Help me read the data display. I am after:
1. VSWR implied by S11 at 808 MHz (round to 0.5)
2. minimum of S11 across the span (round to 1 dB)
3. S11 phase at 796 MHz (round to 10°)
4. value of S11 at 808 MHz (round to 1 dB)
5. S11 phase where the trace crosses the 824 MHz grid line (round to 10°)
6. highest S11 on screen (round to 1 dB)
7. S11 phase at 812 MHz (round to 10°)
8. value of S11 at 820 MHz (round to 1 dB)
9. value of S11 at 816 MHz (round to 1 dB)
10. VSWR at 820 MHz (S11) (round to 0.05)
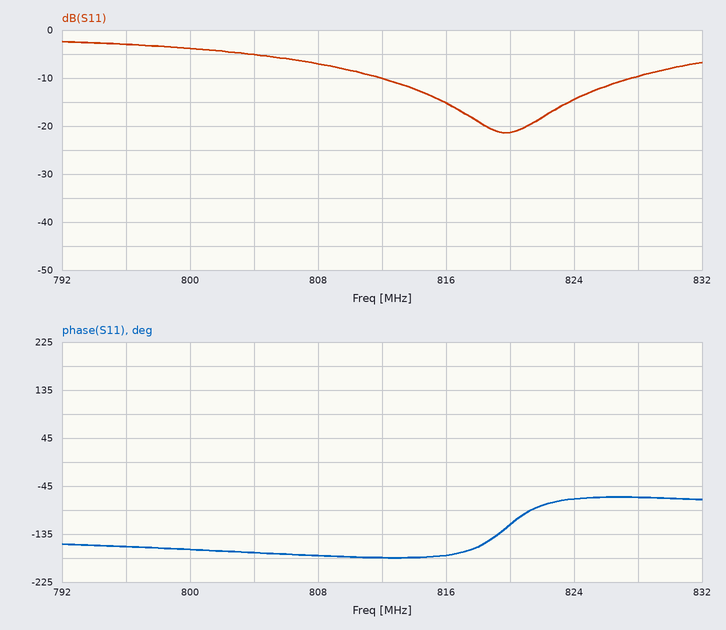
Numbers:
2.5
-21 dB
-160°
-7 dB
-70°
-2 dB
-180°
-21 dB
-15 dB
1.20
